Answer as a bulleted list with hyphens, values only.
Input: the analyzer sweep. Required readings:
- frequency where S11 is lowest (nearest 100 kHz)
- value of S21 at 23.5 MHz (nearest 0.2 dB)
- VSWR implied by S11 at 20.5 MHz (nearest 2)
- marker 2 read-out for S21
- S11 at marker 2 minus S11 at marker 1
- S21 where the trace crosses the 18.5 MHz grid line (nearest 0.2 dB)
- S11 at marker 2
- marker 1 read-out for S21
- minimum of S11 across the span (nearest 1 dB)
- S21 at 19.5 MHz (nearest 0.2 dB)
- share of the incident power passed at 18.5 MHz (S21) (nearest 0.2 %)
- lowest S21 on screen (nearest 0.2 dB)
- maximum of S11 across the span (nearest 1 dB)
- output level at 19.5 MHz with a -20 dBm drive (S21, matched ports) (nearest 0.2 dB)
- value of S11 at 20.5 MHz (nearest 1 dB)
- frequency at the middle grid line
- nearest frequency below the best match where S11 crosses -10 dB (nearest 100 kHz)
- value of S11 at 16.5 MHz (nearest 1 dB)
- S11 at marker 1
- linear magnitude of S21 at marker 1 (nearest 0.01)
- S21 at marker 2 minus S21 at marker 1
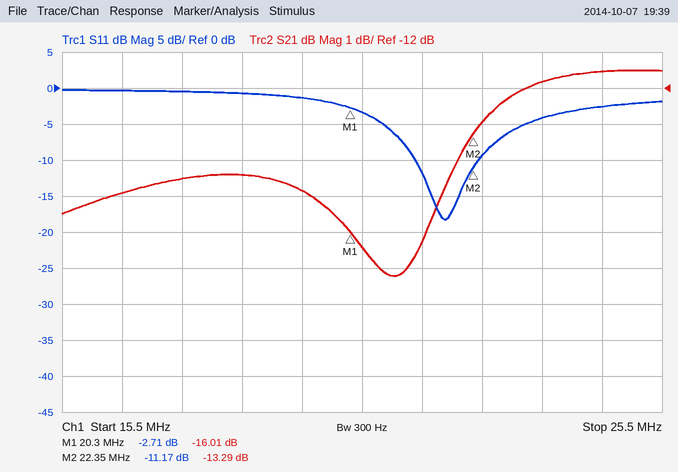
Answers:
- 21.9 MHz
- -11.8 dB
- 6
- -13.29 dB
- -8.46 dB
- -14.4 dB
- -11.17 dB
- -16.01 dB
- -18 dB
- -14.8 dB
- 3.6 %
- -17.2 dB
- 0 dB
- -34.8 dBm
- -3 dB
- 20.5 MHz
- 21.4 MHz
- 0 dB
- -2.71 dB
- 0.16
- 2.72 dB
